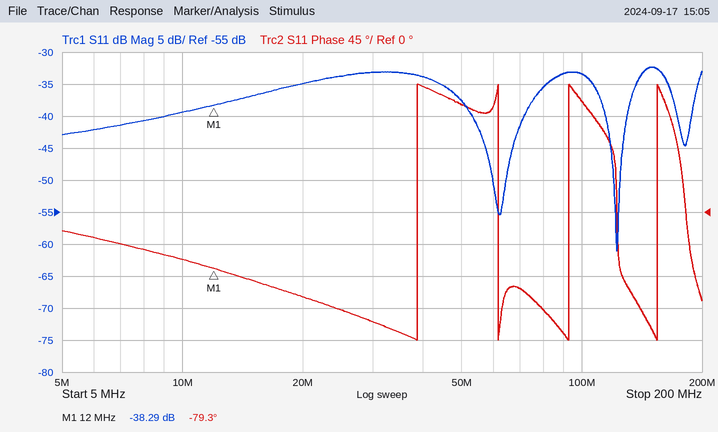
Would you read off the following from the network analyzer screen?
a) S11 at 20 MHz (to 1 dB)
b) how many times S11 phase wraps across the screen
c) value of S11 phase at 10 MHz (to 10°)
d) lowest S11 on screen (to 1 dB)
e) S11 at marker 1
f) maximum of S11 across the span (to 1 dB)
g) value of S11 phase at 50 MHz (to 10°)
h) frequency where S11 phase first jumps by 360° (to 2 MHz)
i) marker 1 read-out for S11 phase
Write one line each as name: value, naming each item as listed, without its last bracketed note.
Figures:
S11 at 20 MHz: -35 dB
how many times S11 phase wraps across the screen: 4
value of S11 phase at 10 MHz: -70°
lowest S11 on screen: -61 dB
S11 at marker 1: -38.29 dB
maximum of S11 across the span: -32 dB
value of S11 phase at 50 MHz: 150°
frequency where S11 phase first jumps by 360°: 38 MHz
marker 1 read-out for S11 phase: -79.3°
